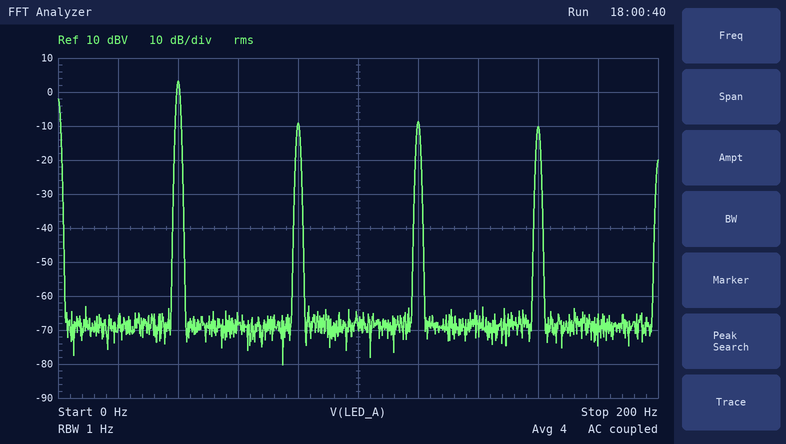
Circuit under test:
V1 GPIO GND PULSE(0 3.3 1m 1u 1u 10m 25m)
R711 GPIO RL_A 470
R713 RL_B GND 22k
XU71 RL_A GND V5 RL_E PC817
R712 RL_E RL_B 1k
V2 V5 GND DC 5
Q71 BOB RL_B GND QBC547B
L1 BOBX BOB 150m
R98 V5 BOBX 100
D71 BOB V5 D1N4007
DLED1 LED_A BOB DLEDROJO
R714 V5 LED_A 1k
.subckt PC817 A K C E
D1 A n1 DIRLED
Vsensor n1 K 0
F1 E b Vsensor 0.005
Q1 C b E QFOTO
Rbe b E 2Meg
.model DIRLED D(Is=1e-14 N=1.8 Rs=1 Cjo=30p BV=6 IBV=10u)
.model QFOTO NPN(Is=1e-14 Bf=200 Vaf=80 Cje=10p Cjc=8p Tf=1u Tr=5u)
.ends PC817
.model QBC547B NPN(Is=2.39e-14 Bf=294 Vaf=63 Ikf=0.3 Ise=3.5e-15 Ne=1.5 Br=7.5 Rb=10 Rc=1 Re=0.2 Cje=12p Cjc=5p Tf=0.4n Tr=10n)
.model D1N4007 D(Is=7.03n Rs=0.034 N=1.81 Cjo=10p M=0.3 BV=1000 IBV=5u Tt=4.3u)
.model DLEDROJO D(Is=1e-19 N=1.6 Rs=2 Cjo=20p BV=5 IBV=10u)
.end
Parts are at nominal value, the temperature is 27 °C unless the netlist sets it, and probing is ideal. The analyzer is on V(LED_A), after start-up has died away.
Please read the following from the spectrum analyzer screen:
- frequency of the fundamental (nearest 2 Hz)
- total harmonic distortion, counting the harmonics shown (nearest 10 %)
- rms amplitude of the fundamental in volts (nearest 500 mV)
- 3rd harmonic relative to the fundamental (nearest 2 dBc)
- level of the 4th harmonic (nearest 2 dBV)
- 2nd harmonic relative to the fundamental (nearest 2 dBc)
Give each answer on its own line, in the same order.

40 Hz
40 %
1.5 V
-12 dBc
-10 dBV
-12 dBc
